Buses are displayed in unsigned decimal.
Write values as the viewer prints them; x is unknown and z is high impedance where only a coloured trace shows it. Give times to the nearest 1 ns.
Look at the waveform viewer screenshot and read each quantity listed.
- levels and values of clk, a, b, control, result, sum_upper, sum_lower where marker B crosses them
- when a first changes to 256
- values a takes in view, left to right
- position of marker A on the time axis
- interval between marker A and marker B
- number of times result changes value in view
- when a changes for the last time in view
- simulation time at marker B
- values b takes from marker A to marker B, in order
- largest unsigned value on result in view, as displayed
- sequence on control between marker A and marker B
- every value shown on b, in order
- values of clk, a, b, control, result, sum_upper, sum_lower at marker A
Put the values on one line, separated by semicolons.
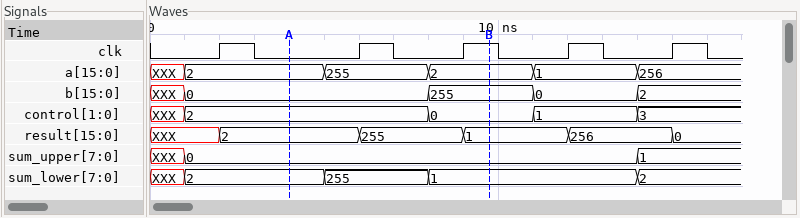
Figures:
clk=1, a=2, b=255, control=0, result=1, sum_upper=0, sum_lower=1; 14 ns; XXX, 2, 255, 2, 1, 256; 4 ns; 6 ns; 5; 14 ns; 10 ns; 0, 255; 256; 2, 0; XXX, 0, 255, 0, 2; clk=0, a=2, b=0, control=2, result=2, sum_upper=0, sum_lower=2
